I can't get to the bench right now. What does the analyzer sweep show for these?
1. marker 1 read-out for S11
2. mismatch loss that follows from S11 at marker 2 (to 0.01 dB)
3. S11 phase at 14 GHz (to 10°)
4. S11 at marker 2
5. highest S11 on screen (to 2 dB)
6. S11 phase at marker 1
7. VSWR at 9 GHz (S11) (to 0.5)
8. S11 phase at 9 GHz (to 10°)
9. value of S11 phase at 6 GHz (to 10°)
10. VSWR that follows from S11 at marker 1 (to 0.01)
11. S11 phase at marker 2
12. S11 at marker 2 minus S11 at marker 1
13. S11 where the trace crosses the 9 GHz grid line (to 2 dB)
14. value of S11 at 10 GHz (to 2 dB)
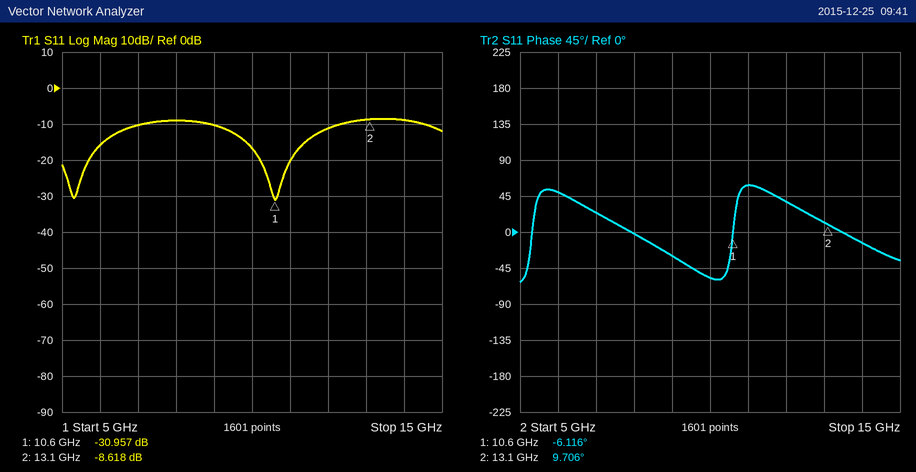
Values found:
-30.957 dB
0.64 dB
-10°
-8.618 dB
-8 dB
-6.116°
2.0
-30°
50°
1.06
9.706°
22.339 dB
-10 dB
-16 dB
